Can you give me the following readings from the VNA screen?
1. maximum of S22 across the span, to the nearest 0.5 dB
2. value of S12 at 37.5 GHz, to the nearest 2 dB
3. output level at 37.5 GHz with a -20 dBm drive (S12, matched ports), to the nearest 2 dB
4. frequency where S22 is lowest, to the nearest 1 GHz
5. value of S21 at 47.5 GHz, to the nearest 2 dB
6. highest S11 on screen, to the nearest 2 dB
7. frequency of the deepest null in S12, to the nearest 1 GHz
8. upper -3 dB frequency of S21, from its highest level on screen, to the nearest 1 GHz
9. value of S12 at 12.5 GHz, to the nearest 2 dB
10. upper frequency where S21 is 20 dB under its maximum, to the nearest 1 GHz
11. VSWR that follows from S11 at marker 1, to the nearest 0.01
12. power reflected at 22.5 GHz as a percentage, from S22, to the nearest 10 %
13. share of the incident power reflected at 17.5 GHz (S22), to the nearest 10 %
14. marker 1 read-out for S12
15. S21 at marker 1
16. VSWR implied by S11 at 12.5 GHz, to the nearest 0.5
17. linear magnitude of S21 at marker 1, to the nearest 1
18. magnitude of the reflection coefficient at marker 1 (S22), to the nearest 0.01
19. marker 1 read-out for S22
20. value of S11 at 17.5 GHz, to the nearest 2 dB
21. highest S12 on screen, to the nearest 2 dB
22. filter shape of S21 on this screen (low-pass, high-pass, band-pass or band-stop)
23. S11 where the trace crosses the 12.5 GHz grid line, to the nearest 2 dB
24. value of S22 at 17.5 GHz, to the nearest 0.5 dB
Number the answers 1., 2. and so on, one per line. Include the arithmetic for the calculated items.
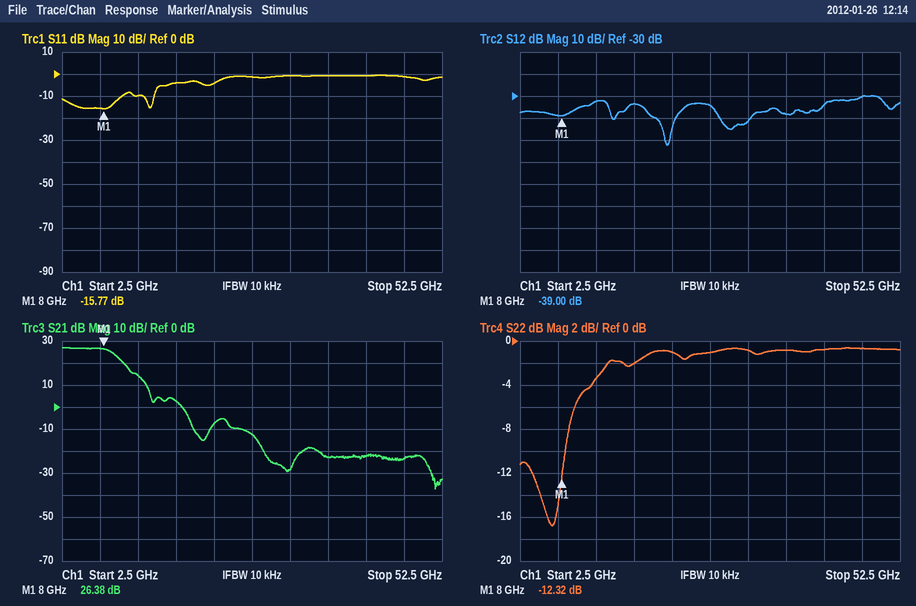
1. -0.5 dB
2. -38 dB
3. -20 dBm + (-38 dB) = -58 dBm
4. 7 GHz
5. -24 dB
6. 0 dB
7. 22 GHz
8. 9 GHz
9. -32 dB
10. 14 GHz
11. (1 + 0.1627)/(1 − 0.1627) ≈ 1.39
12. 10^(-1/10) ≈ 79.4 %, so 80 % to the nearest 10 %
13. 10^(-2/10) ≈ 63.1 %, so 60 % to the nearest 10 %
14. -39.00 dB
15. 26.38 dB
16. |Γ| = 10^(-10/20) = 0.3162; VSWR = (1 + 0.3162)/(1 − 0.3162) ≈ 1.92, so 2.0 to the nearest 0.5
17. 10^(26.38/20) ≈ 21
18. 10^(-12.32/20) ≈ 0.24
19. -12.32 dB
20. -4 dB
21. -30 dB
22. low-pass
23. -10 dB
24. -2.0 dB
